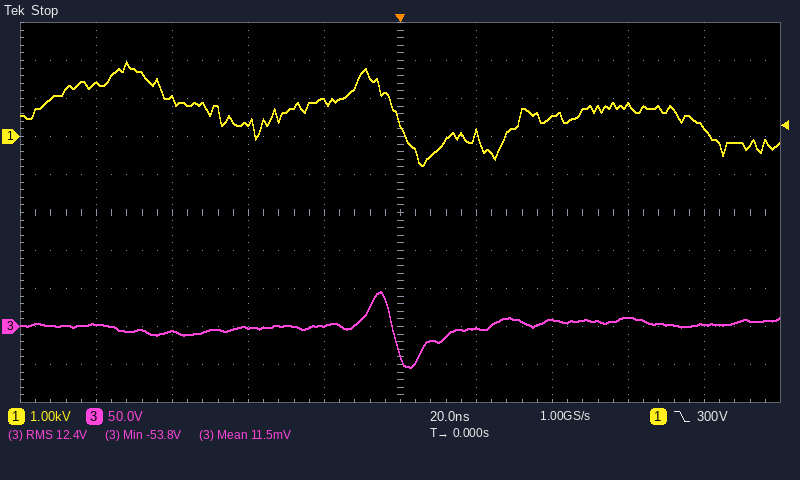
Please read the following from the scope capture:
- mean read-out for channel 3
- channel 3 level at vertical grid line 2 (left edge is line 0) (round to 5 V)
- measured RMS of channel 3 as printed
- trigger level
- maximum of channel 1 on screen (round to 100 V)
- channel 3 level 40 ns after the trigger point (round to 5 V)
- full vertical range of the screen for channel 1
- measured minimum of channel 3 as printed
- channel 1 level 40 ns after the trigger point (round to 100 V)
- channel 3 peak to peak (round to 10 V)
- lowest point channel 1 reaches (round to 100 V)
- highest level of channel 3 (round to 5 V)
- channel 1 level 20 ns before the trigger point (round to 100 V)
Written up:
11.5 mV
-5 V
12.4 V
300 V
2.0 kV
10 V
10 kV
-53.8 V
500 V
100 V
-800 V
45 V
900 V
